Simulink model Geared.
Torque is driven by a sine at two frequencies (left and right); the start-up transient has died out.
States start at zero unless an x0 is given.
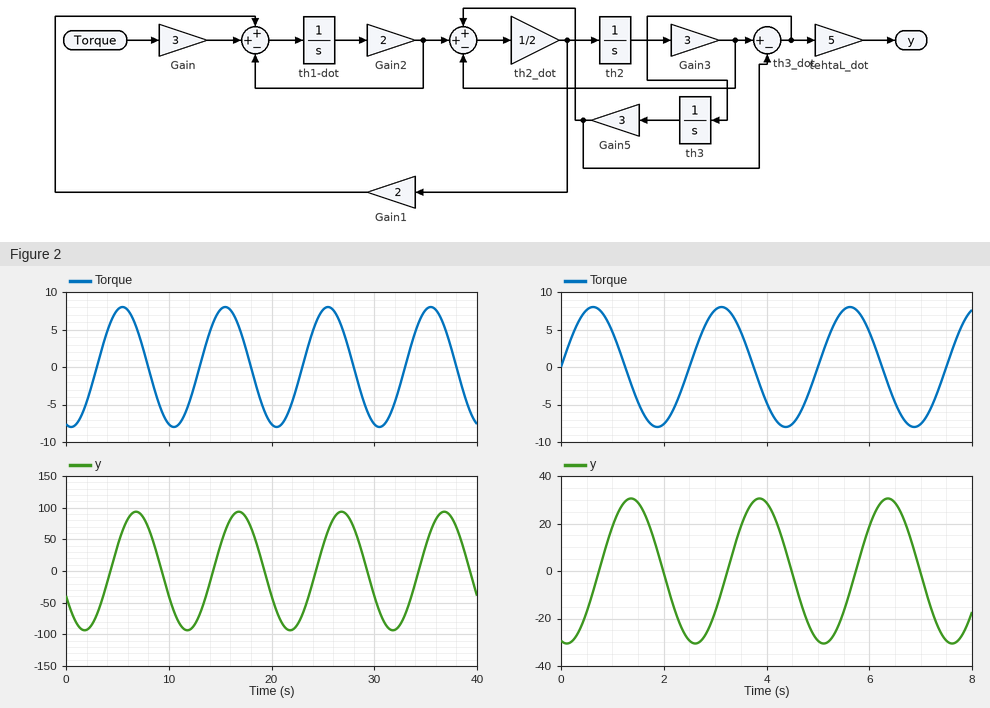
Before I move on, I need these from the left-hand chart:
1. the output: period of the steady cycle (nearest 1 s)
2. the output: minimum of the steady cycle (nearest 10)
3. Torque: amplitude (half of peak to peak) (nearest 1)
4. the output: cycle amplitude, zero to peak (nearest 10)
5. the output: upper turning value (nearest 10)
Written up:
10 s
-90
8
90
90
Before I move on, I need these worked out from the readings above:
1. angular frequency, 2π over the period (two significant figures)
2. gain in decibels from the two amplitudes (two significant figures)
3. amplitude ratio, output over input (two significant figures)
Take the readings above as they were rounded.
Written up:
0.63 rad/s
21 dB
11
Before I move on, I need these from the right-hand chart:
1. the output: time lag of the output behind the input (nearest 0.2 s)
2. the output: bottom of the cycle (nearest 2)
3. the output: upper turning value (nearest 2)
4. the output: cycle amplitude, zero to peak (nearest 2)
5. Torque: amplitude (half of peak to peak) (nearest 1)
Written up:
0.8 s
-30
30
30
8
